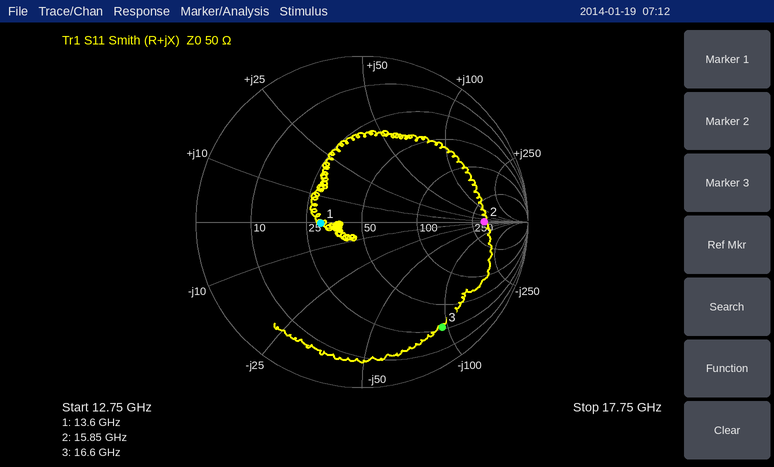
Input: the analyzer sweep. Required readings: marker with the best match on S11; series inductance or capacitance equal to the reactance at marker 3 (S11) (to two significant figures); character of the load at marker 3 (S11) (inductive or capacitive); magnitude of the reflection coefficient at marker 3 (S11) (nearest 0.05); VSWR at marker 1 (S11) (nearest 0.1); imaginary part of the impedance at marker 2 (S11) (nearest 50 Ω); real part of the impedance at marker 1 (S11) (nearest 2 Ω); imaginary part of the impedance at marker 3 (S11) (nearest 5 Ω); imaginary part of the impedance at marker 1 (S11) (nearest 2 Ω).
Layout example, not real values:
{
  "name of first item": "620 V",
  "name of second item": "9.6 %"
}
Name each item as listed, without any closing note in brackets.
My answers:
{
  "marker with the best match on S11": "marker 1",
  "series inductance or capacitance equal to the reactance at marker 3 (S11)": "100 fF",
  "character of the load at marker 3 (S11)": "capacitive",
  "magnitude of the reflection coefficient at marker 3 (S11)": "0.80",
  "VSWR at marker 1 (S11)": "1.7",
  "imaginary part of the impedance at marker 2 (S11)": "0 Ω",
  "real part of the impedance at marker 1 (S11)": "30 Ω",
  "imaginary part of the impedance at marker 3 (S11)": "-95 Ω",
  "imaginary part of the impedance at marker 1 (S11)": "0 Ω"
}
